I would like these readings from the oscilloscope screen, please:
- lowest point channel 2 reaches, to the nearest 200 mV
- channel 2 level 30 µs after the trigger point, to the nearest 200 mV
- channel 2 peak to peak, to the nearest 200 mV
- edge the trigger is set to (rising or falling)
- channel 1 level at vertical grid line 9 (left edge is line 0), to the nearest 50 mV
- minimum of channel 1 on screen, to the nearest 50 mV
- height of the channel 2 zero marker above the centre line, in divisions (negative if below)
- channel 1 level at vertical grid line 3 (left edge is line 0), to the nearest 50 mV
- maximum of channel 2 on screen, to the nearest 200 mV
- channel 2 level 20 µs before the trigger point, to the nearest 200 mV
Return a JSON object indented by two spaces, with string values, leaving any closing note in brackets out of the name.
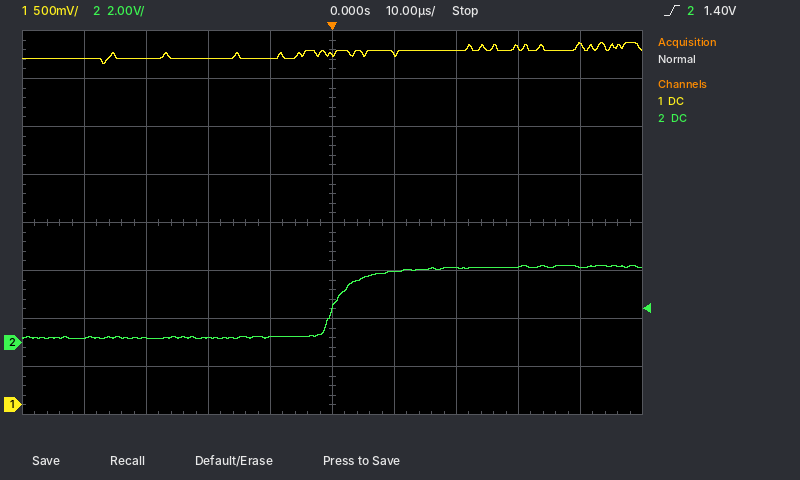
{
  "lowest point channel 2 reaches, to the nearest 200 mV": "200 mV",
  "channel 2 level 30 µs after the trigger point, to the nearest 200 mV": "3.2 V",
  "channel 2 peak to peak, to the nearest 200 mV": "3.0 V",
  "edge the trigger is set to": "rising",
  "channel 1 level at vertical grid line 9 (left edge is line 0), to the nearest 50 mV": "3.75 V",
  "minimum of channel 1 on screen, to the nearest 50 mV": "3.55 V",
  "height of the channel 2 zero marker above the centre line, in divisions": "-2.5 div",
  "channel 1 level at vertical grid line 3 (left edge is line 0), to the nearest 50 mV": "3.60 V",
  "maximum of channel 2 on screen, to the nearest 200 mV": "3.2 V",
  "channel 2 level 20 µs before the trigger point, to the nearest 200 mV": "200 mV"
}
